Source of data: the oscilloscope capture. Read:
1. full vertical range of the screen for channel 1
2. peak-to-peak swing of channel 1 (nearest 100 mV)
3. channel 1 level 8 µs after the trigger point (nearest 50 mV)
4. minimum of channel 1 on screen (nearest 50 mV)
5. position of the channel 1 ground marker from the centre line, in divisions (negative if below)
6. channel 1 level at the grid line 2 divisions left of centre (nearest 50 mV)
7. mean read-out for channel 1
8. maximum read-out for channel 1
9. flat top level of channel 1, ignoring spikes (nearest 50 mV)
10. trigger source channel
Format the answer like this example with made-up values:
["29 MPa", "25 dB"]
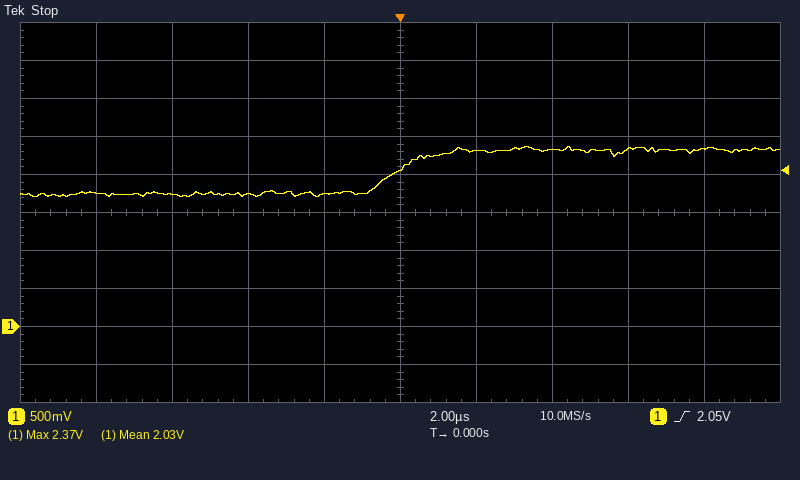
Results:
["5 V", "700 mV", "2.35 V", "1.70 V", "-3.0 div", "1.75 V", "2.03 V", "2.37 V", "2.35 V", "channel 1"]
